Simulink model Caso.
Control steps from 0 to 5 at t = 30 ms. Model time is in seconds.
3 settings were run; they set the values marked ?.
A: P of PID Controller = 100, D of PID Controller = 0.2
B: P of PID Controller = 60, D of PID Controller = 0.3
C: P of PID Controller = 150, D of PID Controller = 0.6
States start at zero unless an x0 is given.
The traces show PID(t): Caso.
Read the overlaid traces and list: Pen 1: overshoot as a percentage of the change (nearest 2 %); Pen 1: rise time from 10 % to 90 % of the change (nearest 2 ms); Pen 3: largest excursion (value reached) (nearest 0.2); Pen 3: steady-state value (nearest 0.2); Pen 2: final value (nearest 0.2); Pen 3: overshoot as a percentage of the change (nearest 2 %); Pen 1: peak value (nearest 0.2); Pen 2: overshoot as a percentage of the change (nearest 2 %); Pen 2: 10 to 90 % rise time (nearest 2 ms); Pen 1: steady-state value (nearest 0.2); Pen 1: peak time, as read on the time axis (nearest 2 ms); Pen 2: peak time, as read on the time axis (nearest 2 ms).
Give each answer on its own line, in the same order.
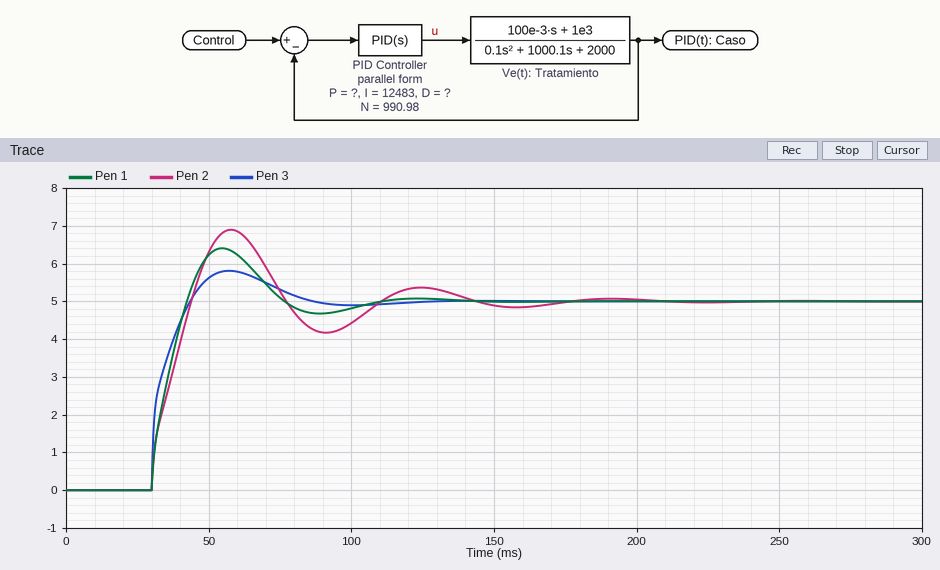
28 %
10 ms
5.8
5.0
5.0
16 %
6.4
38 %
12 ms
5.0
54 ms
58 ms
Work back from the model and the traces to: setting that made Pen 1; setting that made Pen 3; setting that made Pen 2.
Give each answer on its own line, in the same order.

A
C
B
